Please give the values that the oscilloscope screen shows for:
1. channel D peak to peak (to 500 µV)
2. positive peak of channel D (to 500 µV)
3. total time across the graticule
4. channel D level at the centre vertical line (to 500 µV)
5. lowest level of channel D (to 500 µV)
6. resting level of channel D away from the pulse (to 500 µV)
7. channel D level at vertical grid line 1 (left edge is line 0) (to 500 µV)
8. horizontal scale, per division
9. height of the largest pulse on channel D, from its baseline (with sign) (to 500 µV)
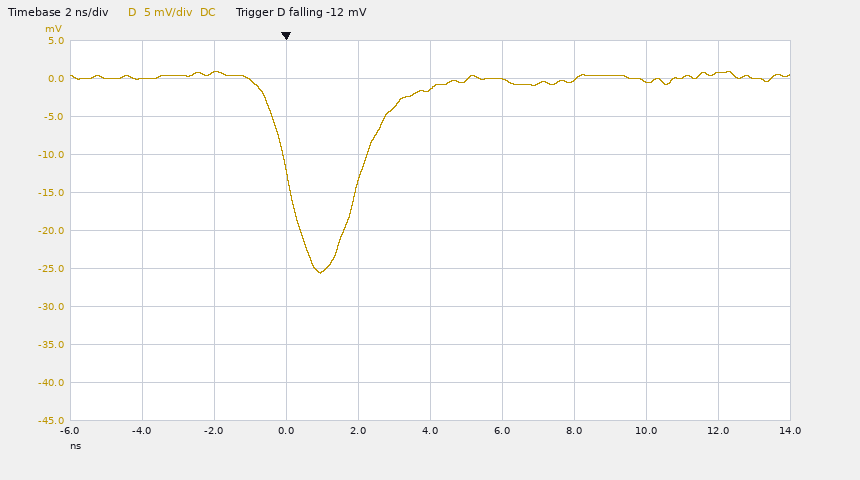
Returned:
26.5 mV
1.0 mV
20 ns
-1.5 mV
-25.5 mV
0.0 mV
0.0 mV
2 ns
-25.5 mV
